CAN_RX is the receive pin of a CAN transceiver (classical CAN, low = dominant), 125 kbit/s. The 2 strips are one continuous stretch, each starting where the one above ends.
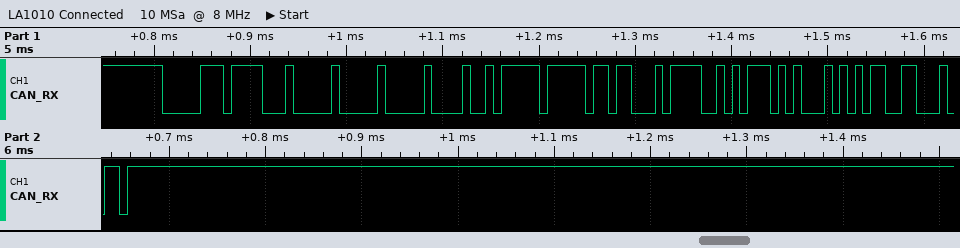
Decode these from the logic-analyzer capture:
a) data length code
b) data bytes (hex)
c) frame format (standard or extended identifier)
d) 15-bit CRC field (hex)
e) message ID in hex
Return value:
8
00 00 97 FF B1 79 5D 45
standard
0x2CC5
0x06F
